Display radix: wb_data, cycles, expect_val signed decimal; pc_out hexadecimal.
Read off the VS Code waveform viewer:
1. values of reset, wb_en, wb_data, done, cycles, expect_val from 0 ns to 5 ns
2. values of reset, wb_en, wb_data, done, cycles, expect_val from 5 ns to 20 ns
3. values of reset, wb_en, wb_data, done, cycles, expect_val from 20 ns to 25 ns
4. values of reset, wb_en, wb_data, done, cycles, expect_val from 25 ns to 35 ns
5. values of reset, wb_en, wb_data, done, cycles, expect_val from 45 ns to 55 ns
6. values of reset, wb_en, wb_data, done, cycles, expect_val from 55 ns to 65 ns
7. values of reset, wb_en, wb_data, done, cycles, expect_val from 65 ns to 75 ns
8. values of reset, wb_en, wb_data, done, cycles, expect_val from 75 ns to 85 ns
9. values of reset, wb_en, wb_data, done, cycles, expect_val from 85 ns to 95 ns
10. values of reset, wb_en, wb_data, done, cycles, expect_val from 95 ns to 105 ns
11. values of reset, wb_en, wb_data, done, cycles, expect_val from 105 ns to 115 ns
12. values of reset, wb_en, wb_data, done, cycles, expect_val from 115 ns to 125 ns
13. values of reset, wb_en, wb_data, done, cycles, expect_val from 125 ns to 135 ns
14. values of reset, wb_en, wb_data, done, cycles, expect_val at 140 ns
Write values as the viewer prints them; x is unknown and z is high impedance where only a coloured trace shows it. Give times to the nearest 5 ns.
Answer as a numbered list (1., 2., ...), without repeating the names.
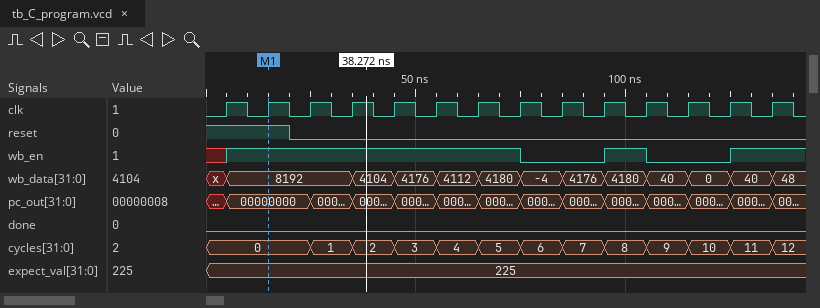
1. reset=1, wb_en=x, wb_data=x, done=0, cycles=0, expect_val=225
2. reset=1, wb_en=1, wb_data=8192, done=0, cycles=0, expect_val=225
3. reset=0, wb_en=1, wb_data=8192, done=0, cycles=0, expect_val=225
4. reset=0, wb_en=1, wb_data=8192, done=0, cycles=1, expect_val=225
5. reset=0, wb_en=1, wb_data=4176, done=0, cycles=3, expect_val=225
6. reset=0, wb_en=1, wb_data=4112, done=0, cycles=4, expect_val=225
7. reset=0, wb_en=1, wb_data=4180, done=0, cycles=5, expect_val=225
8. reset=0, wb_en=0, wb_data=-4, done=0, cycles=6, expect_val=225
9. reset=0, wb_en=0, wb_data=4176, done=0, cycles=7, expect_val=225
10. reset=0, wb_en=1, wb_data=4180, done=0, cycles=8, expect_val=225
11. reset=0, wb_en=0, wb_data=40, done=0, cycles=9, expect_val=225
12. reset=0, wb_en=0, wb_data=0, done=0, cycles=10, expect_val=225
13. reset=0, wb_en=1, wb_data=40, done=0, cycles=11, expect_val=225
14. reset=0, wb_en=1, wb_data=48, done=0, cycles=12, expect_val=225
